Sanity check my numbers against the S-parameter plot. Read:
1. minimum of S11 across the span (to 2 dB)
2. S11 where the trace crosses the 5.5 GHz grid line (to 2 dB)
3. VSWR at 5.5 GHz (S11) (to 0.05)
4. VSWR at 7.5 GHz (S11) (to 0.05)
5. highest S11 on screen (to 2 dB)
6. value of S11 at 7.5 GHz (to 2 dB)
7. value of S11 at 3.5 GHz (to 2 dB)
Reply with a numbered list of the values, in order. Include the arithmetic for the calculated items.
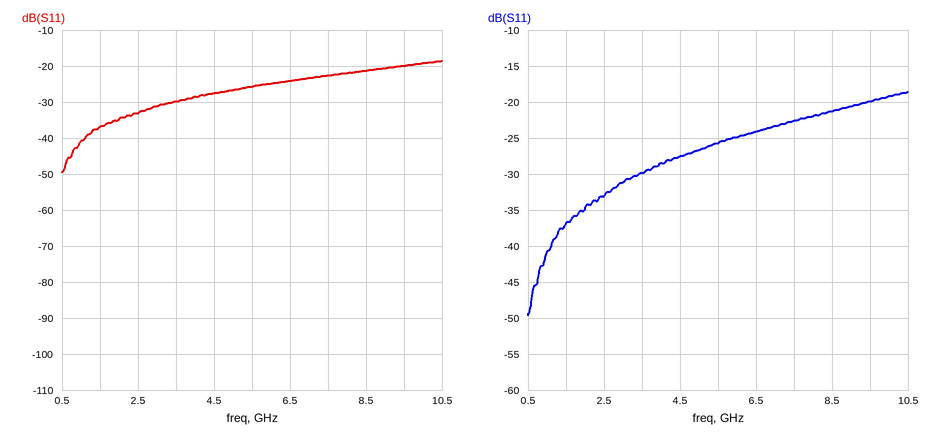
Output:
1. -50 dB
2. -26 dB
3. |Γ| = 10^(-26/20) = 0.0501; VSWR = (1 + 0.0501)/(1 − 0.0501) ≈ 1.11, so 1.10 to the nearest 0.05
4. |Γ| = 10^(-22/20) = 0.0794; VSWR = (1 + 0.0794)/(1 − 0.0794) ≈ 1.17, so 1.15 to the nearest 0.05
5. -18 dB
6. -22 dB
7. -30 dB
